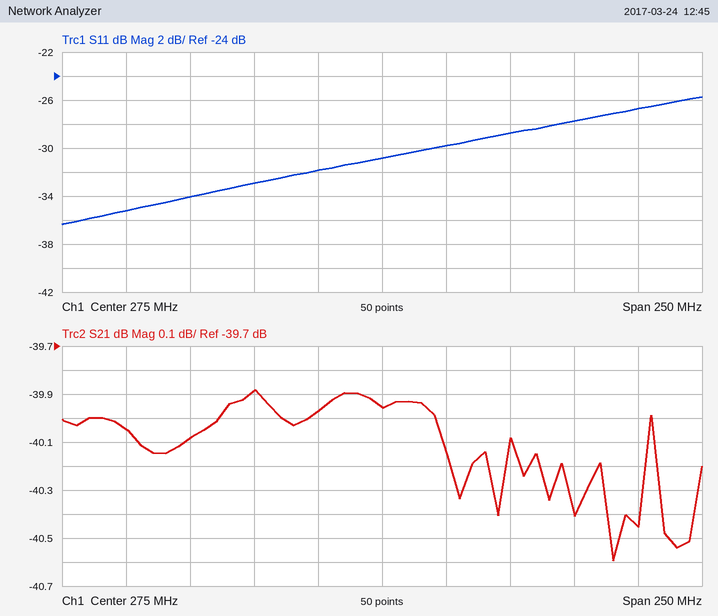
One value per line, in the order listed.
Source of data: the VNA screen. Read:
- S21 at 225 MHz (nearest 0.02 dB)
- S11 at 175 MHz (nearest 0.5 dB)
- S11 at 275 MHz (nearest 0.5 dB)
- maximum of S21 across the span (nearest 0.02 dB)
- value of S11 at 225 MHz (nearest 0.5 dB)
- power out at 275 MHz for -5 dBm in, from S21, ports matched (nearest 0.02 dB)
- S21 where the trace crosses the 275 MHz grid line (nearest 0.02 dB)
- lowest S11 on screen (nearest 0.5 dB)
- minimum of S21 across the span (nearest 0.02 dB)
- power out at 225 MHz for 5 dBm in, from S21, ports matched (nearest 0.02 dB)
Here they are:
-39.88 dB
-35.0 dB
-31.0 dB
-39.88 dB
-33.0 dB
-44.96 dBm
-39.96 dB
-36.5 dB
-40.60 dB
-34.88 dBm
